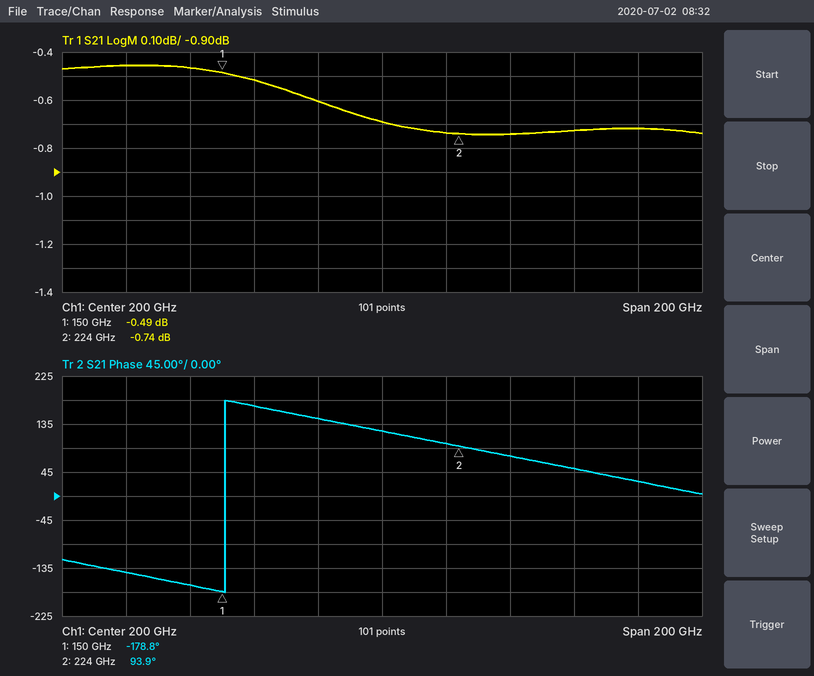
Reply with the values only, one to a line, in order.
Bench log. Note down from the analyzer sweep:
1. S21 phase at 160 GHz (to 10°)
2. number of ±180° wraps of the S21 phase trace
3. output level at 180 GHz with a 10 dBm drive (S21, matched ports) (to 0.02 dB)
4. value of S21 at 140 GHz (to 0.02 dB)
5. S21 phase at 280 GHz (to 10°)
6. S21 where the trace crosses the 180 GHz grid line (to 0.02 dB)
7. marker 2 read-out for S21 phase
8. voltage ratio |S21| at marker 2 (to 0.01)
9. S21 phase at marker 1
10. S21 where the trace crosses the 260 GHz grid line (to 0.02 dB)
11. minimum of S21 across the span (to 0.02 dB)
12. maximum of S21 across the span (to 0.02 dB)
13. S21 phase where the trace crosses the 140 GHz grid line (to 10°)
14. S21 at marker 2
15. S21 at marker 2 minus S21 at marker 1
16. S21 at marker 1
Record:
170°
1
9.40 dBm
-0.46 dB
30°
-0.60 dB
93.9°
0.92
-178.8°
-0.72 dB
-0.74 dB
-0.46 dB
-170°
-0.74 dB
-0.25 dB
-0.49 dB
